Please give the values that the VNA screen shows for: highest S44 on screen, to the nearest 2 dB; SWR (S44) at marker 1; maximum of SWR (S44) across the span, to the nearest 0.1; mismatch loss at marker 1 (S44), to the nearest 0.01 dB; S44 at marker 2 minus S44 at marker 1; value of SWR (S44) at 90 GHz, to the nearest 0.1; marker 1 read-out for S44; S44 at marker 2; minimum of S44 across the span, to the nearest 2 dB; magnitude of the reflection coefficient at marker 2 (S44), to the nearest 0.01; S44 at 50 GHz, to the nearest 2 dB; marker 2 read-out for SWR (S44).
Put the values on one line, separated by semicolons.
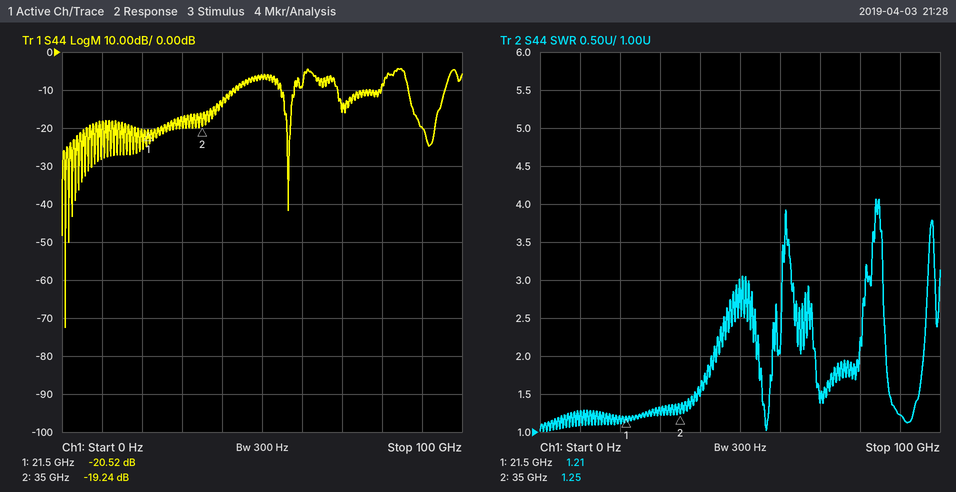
-4 dB; 1.21; 4.1; 0.04 dB; 1.28 dB; 1.2; -20.52 dB; -19.24 dB; -72 dB; 0.11; -6 dB; 1.25
